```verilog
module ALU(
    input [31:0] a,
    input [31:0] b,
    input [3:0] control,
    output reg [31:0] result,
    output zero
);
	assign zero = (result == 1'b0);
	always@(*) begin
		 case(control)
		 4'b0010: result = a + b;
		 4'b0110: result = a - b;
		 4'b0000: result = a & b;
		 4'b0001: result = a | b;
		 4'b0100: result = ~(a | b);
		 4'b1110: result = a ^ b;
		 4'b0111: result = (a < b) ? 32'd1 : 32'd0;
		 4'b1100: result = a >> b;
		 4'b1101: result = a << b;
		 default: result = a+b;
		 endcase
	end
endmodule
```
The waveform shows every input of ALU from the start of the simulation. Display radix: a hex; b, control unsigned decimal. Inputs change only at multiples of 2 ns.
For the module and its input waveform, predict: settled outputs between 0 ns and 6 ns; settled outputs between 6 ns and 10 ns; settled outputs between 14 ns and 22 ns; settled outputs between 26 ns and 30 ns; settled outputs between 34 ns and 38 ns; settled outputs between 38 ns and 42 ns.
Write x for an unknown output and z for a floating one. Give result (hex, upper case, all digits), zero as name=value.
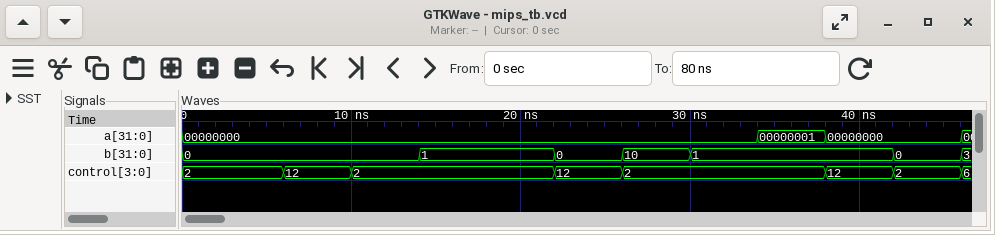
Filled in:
result=00000000, zero=1
result=00000000, zero=1
result=00000001, zero=0
result=0000000A, zero=0
result=00000002, zero=0
result=00000000, zero=1
